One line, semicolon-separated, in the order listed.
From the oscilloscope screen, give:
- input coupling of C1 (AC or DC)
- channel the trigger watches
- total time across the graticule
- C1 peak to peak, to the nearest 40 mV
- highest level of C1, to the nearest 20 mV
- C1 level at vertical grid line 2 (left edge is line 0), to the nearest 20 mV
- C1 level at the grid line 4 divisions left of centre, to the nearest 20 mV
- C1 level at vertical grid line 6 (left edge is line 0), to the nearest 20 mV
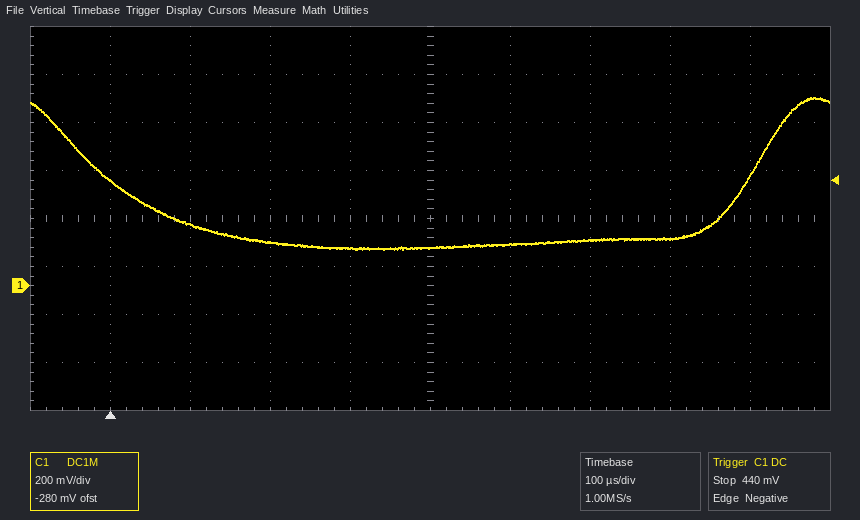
DC; C1; 1 ms; 640 mV; 780 mV; 260 mV; 440 mV; 180 mV
